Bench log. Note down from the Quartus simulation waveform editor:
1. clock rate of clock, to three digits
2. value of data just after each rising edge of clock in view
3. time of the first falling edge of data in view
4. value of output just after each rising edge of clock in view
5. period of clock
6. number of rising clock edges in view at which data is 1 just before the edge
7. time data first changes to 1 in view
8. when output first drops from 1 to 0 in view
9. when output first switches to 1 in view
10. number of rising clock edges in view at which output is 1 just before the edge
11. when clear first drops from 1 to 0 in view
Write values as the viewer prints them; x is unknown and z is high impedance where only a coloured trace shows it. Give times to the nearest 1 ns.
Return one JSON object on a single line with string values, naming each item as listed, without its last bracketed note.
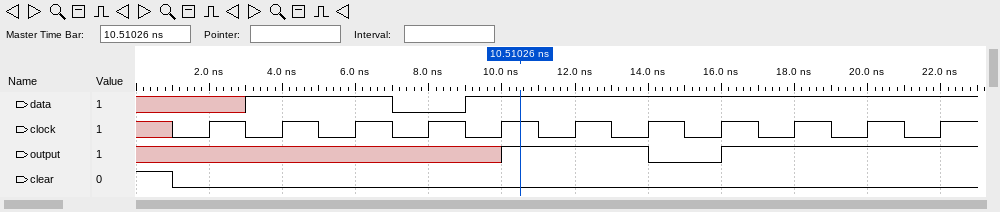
{"clock rate of clock, to three digits": "500 MHz", "value of data just after each rising edge of clock in view": "x 1 1 0 1 1 1 1 1 1 1", "time of the first falling edge of data in view": "7 ns", "value of output just after each rising edge of clock in view": "x x x x 1 1 0 1 1 1 1", "period of clock": "2 ns", "number of rising clock edges in view at which data is 1 just before the edge": "9", "time data first changes to 1 in view": "3 ns", "when output first drops from 1 to 0 in view": "14 ns", "when output first switches to 1 in view": "10 ns", "number of rising clock edges in view at which output is 1 just before the edge": "5", "when clear first drops from 1 to 0 in view": "1 ns"}
